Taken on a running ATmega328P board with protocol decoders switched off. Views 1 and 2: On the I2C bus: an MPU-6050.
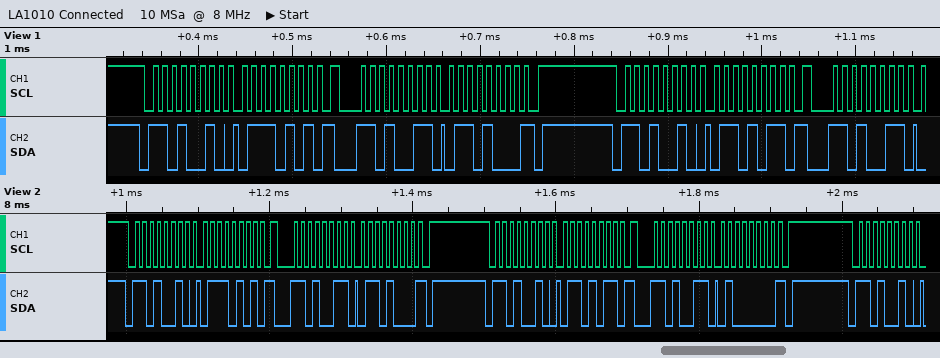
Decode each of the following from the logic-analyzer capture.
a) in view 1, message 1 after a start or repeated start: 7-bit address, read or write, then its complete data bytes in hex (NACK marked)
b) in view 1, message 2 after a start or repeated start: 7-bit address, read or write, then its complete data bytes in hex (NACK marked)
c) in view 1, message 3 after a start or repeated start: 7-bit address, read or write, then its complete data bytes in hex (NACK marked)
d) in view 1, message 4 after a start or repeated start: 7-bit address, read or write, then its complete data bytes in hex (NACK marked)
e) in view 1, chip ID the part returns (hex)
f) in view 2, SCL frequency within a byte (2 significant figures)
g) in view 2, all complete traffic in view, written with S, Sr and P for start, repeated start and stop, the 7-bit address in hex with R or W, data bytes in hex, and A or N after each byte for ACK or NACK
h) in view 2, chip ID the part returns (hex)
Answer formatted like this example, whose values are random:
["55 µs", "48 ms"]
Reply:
["0x69 write: 75", "0x69 read: 68 NACK", "0x69 write: 6B", "0x69 read", "0x68", "100 kHz", "S 69W A 75 A Sr 69R A 68 N P S 69W A 6B A Sr 69R A 40 N P S 69W A", "0x68"]
